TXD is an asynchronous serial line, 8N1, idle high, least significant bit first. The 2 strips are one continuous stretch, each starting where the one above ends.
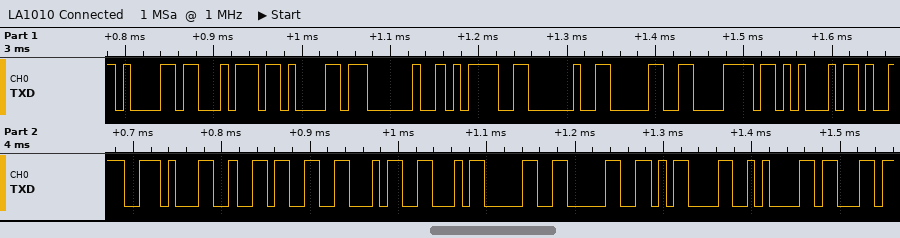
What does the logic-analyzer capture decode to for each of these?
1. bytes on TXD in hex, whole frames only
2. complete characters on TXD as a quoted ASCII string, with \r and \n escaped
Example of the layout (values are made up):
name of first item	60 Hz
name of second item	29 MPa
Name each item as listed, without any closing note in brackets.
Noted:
bytes on TXD in hex, whole frames only	0x61 0x74 0x61 0x20 0x3D 0x20 0x30 0x78 0x45 0x39 0x31 0x36 0x46 0x46 0x30 0x30 0x0D 0x0A 0x63
complete characters on TXD as a quoted ASCII string, with \r and \n escaped	"ata = 0xE916FF00\r\nc"
